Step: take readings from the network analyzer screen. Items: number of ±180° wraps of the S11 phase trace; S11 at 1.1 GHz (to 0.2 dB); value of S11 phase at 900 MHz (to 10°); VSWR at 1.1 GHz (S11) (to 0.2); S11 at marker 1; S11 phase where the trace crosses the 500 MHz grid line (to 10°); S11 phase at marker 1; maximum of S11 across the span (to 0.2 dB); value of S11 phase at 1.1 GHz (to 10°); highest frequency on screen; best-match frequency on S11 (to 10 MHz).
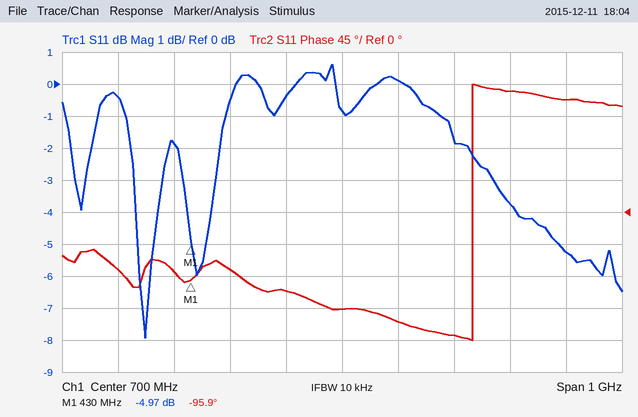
1
-5.2 dB
-170°
3.4
-4.97 dB
-80°
-95.9°
0.6 dB
160°
1.2 GHz
350 MHz
